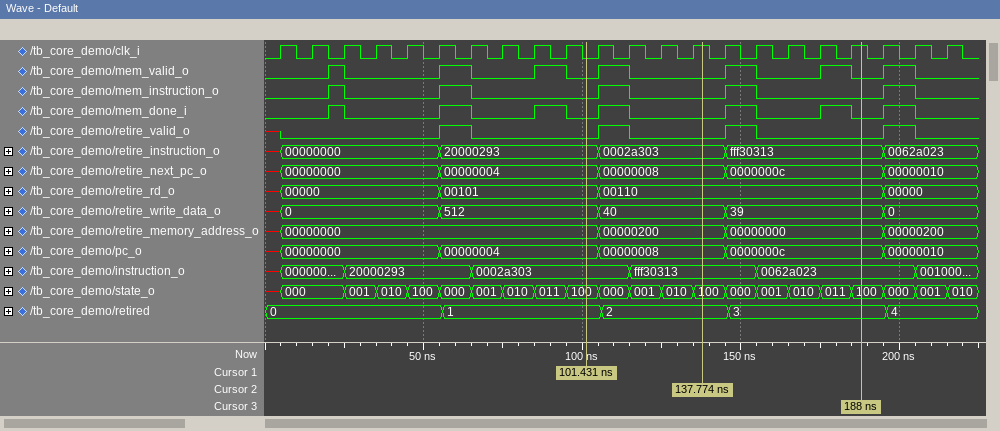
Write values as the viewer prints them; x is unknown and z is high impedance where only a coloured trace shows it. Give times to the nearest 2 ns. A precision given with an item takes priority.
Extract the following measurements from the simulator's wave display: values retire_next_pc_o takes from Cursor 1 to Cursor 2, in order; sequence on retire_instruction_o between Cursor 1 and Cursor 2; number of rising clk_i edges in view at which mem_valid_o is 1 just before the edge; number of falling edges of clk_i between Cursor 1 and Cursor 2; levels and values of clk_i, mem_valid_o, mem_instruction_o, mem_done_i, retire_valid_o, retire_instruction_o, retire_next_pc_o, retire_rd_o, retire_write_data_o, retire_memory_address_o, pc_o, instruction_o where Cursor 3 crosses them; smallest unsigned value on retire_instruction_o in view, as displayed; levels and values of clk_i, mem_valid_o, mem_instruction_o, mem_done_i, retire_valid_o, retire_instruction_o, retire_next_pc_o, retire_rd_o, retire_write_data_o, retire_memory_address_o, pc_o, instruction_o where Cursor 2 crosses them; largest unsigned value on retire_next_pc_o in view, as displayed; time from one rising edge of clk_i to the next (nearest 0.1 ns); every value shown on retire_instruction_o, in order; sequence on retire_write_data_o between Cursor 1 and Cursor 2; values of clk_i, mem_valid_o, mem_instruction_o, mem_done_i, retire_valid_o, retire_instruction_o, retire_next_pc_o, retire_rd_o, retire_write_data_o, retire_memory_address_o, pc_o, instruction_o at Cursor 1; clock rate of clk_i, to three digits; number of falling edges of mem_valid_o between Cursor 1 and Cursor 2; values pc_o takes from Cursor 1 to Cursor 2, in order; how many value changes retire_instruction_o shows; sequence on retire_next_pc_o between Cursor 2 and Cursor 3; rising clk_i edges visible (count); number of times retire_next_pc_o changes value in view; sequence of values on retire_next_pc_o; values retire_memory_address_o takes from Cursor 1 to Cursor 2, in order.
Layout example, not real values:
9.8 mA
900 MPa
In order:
00000004, 00000008
20000293, 0002a303
7
3
clk_i=1, mem_valid_o=0, mem_instruction_o=0, mem_done_i=0, retire_valid_o=0, retire_instruction_o=fff30313, retire_next_pc_o=0000000c, retire_rd_o=00110, retire_write_data_o=39, retire_memory_address_o=00000000, pc_o=0000000c, instruction_o=0062a023
00000000
clk_i=1, mem_valid_o=0, mem_instruction_o=0, mem_done_i=0, retire_valid_o=0, retire_instruction_o=0002a303, retire_next_pc_o=00000008, retire_rd_o=00110, retire_write_data_o=40, retire_memory_address_o=00000200, pc_o=00000008, instruction_o=fff30313
00000010
10 ns
x, 00000000, 20000293, 0002a303, fff30313, 0062a023
512, 40
clk_i=0, mem_valid_o=0, mem_instruction_o=0, mem_done_i=0, retire_valid_o=0, retire_instruction_o=20000293, retire_next_pc_o=00000004, retire_rd_o=00101, retire_write_data_o=512, retire_memory_address_o=00000000, pc_o=00000004, instruction_o=0002a303
100 MHz
1
00000004, 00000008
5
00000008, 0000000c
22
5
x, 00000000, 00000004, 00000008, 0000000c, 00000010
00000000, 00000200
